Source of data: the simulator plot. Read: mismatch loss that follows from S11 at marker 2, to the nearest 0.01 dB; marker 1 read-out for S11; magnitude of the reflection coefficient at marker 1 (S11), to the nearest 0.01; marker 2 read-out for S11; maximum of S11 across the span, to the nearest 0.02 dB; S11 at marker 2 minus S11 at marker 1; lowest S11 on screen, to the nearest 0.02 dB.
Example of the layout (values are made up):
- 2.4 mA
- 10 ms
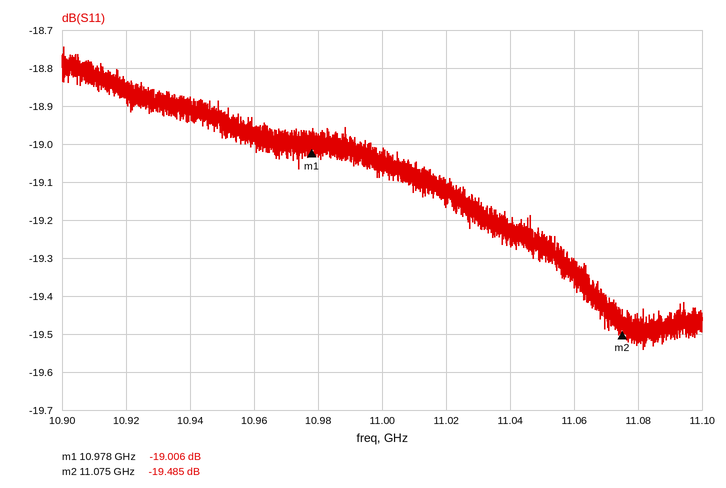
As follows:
- 0.05 dB
- -19.006 dB
- 0.11
- -19.485 dB
- -18.74 dB
- -0.479 dB
- -19.54 dB
